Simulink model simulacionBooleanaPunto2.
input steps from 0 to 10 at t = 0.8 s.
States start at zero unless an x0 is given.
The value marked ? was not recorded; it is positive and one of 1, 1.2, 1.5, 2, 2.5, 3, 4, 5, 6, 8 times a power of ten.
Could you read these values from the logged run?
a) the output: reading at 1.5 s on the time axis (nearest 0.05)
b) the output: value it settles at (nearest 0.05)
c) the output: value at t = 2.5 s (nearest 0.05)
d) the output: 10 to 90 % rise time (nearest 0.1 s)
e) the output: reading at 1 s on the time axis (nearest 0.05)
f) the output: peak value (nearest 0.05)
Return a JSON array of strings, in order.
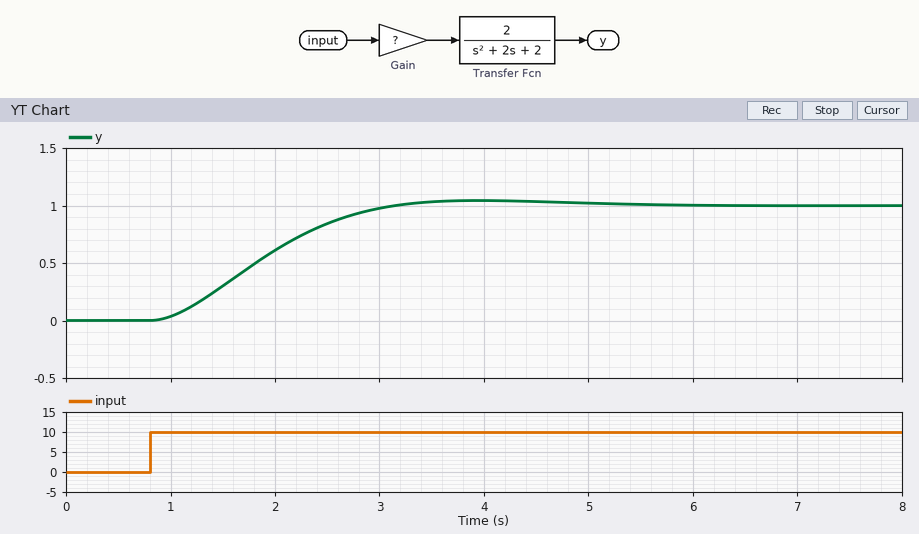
["0.30", "1.00", "0.85", "1.5 s", "0.05", "1.05"]
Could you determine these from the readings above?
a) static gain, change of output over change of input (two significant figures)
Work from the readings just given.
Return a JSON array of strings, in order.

["0.10"]
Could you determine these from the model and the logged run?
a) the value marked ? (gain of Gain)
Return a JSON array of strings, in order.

["0.1"]
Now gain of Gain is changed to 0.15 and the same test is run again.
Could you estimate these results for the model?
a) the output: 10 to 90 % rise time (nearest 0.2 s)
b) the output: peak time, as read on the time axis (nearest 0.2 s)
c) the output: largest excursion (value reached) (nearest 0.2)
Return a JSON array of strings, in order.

["1.6 s", "4.0 s", "1.6"]
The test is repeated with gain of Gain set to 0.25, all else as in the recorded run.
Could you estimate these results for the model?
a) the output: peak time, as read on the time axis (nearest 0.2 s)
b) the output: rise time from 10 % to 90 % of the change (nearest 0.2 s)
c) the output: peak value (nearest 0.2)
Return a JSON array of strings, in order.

["4.0 s", "1.6 s", "2.6"]
